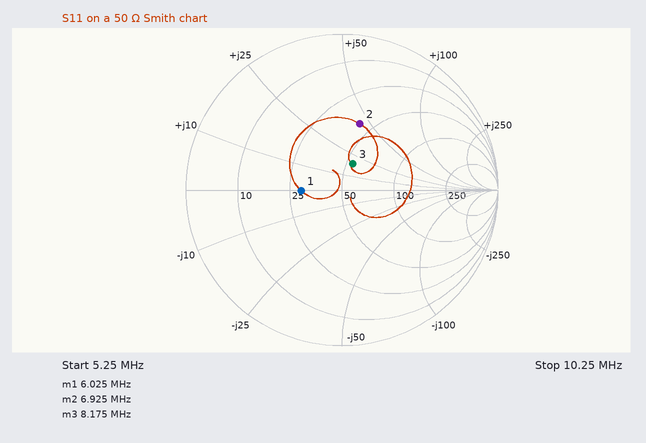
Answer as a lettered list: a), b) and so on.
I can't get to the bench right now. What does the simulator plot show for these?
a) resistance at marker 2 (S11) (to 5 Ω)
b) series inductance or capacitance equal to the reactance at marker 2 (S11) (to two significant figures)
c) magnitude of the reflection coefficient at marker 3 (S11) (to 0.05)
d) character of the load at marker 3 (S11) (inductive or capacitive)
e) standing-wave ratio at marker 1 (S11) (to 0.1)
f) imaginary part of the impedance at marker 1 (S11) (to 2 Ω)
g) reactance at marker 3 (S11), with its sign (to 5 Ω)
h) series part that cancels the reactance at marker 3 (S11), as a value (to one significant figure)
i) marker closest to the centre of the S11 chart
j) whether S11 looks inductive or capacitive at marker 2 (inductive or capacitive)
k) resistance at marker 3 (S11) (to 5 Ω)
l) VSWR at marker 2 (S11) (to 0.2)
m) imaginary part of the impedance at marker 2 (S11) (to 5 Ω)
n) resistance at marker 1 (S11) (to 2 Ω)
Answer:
a) 40 Ω
b) 1.0 µH
c) 0.20
d) inductive
e) 1.7
f) 0 Ω
g) +20 Ω
h) 1 nF
i) marker 3
j) inductive
k) 55 Ω
l) 2.6
m) +45 Ω
n) 30 Ω
